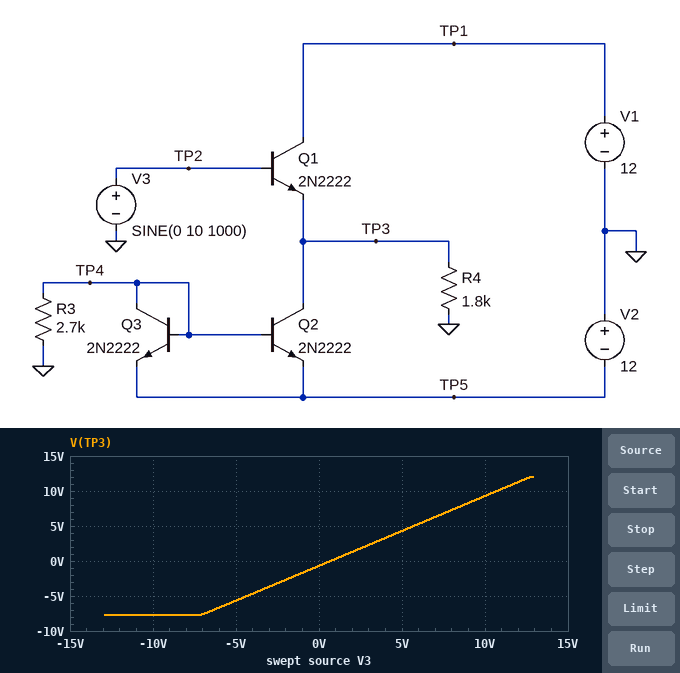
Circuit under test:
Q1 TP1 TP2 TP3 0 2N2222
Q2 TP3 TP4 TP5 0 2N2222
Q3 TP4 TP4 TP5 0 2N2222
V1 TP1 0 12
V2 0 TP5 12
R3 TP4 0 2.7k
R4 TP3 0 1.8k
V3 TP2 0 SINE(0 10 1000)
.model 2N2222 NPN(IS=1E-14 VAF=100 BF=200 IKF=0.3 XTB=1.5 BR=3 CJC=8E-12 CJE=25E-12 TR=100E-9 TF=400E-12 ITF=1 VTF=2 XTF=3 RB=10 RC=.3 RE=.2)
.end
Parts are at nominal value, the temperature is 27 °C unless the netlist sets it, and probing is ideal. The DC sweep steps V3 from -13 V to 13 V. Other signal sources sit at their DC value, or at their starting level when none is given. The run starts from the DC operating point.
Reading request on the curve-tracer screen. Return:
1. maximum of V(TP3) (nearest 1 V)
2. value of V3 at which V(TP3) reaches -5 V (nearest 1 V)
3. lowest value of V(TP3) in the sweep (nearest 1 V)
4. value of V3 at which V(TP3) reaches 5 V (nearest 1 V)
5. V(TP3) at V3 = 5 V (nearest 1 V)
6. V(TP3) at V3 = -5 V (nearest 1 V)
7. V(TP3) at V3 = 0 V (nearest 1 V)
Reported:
12 V
-4 V
-8 V
6 V
4 V
-6 V
-1 V
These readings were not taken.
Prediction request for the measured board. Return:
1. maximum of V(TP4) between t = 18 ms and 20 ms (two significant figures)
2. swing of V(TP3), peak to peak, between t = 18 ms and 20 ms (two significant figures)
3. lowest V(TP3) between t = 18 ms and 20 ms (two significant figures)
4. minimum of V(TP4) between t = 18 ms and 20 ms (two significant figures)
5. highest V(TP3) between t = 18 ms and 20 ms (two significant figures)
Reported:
-11 V
17 V
-7.7 V
-11 V
9.3 V
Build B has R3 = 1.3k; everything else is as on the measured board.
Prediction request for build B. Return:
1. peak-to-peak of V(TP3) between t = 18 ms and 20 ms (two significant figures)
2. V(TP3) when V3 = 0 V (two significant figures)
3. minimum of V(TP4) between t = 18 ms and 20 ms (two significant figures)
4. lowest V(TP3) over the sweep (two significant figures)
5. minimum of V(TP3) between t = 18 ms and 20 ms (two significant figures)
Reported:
20 V
-710 mV
-11 V
-12 V
-11 V
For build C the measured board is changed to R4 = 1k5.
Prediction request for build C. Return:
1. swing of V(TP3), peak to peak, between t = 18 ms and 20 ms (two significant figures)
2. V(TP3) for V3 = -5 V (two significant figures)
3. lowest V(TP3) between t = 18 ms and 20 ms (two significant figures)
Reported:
16 V
-5.6 V
-6.5 V
